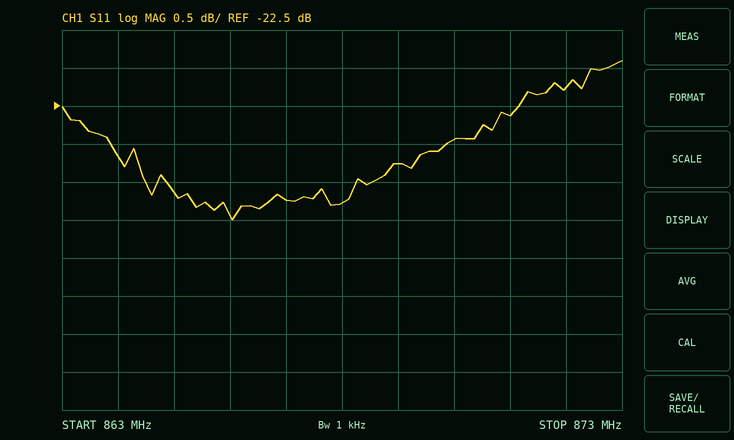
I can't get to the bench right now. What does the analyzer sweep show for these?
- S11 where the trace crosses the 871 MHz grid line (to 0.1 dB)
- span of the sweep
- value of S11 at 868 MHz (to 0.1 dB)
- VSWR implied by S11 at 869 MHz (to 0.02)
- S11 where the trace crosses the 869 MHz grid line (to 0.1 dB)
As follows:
-22.6 dB
10 MHz
-23.8 dB
1.14
-23.3 dB
